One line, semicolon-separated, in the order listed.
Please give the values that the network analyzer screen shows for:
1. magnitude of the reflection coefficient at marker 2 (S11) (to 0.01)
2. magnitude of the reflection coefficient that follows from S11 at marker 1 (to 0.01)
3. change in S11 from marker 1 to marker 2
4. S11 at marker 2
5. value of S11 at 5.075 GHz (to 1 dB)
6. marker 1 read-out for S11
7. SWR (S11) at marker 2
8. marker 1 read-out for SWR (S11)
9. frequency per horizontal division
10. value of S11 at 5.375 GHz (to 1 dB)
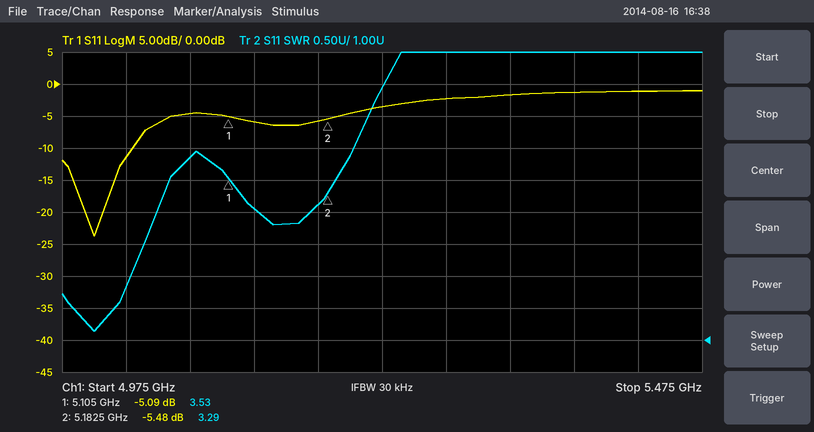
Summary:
0.53; 0.56; -0.39 dB; -5.48 dB; -5 dB; -5.09 dB; 3.29; 3.53; 50 MHz; -1 dB
